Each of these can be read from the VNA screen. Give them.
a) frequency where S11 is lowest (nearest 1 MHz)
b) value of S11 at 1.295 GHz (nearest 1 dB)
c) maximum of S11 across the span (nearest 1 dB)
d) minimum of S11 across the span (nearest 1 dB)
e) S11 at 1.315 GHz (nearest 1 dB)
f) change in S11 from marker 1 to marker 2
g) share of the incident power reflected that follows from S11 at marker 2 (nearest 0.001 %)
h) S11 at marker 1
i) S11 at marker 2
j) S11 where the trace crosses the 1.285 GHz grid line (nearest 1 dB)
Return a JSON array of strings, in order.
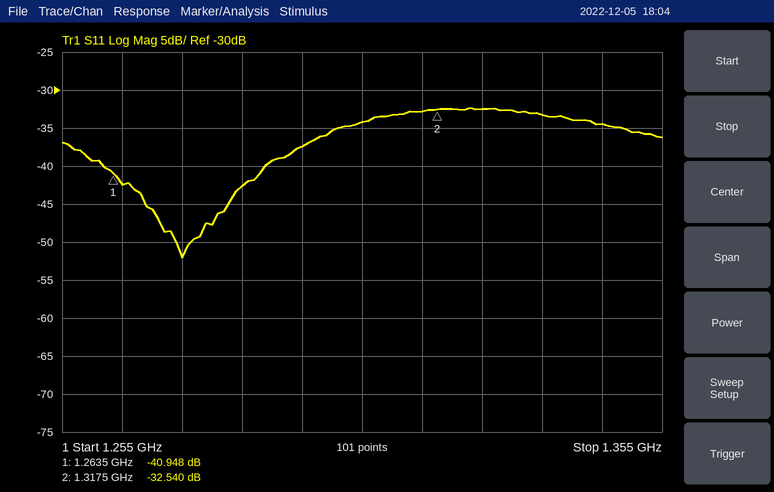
["1.275 GHz", "-37 dB", "-32 dB", "-52 dB", "-33 dB", "8.408 dB", "0.056 %", "-40.948 dB", "-32.540 dB", "-43 dB"]
